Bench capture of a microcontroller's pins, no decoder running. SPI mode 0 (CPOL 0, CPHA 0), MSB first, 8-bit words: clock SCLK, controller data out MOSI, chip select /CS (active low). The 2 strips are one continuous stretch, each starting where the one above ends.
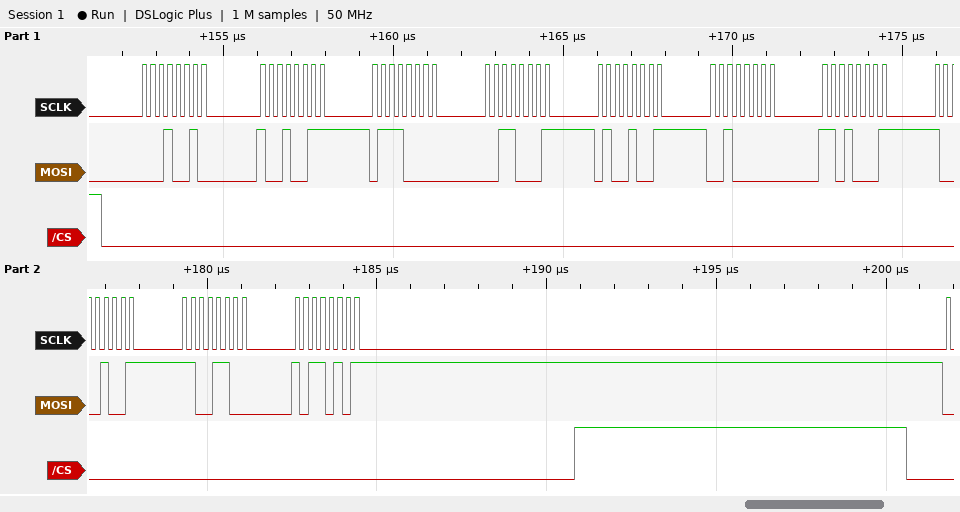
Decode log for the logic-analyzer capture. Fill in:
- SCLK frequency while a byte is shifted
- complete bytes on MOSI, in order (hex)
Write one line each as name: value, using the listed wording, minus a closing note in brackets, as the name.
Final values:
SCLK frequency while a byte is shifted: 4 MHz
complete bytes on MOSI, in order: 12 93 70 31 49 20 D1 89 CC B5
